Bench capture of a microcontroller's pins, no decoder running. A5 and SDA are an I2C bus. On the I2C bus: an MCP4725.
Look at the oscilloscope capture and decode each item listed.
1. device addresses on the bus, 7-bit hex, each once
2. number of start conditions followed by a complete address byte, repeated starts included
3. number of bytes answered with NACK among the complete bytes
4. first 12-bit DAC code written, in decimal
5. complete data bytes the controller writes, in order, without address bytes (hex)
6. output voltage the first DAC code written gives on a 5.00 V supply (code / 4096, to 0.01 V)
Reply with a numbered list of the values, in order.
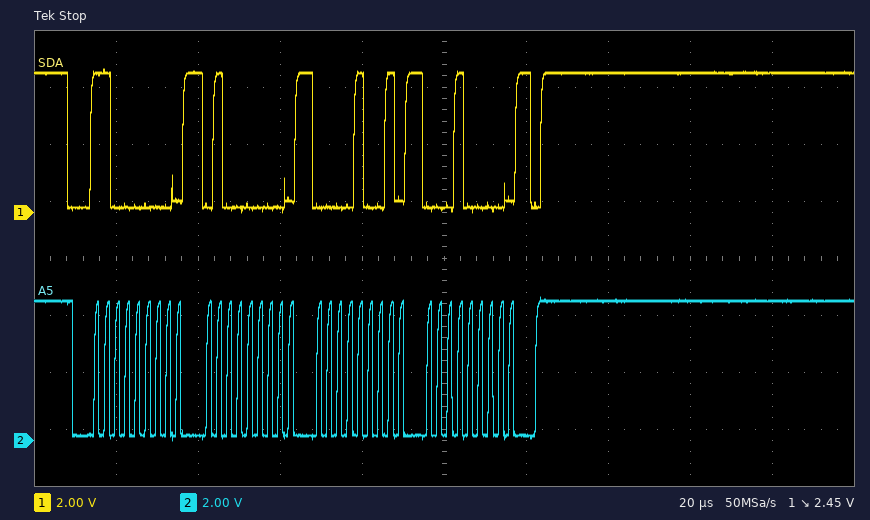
1. 0x60
2. 1
3. 0
4. 145
5. 40 09 10
6. 0.18 V
